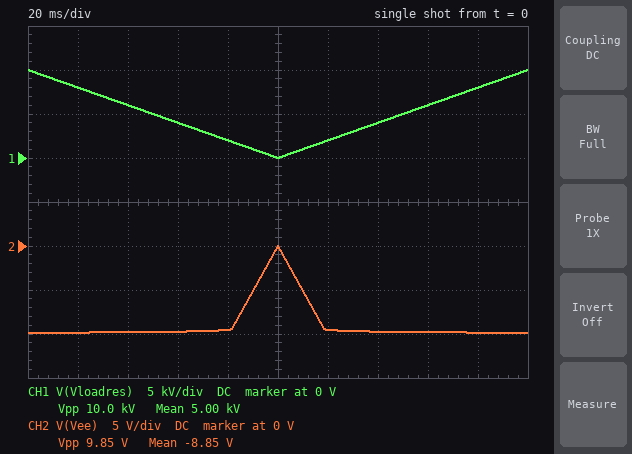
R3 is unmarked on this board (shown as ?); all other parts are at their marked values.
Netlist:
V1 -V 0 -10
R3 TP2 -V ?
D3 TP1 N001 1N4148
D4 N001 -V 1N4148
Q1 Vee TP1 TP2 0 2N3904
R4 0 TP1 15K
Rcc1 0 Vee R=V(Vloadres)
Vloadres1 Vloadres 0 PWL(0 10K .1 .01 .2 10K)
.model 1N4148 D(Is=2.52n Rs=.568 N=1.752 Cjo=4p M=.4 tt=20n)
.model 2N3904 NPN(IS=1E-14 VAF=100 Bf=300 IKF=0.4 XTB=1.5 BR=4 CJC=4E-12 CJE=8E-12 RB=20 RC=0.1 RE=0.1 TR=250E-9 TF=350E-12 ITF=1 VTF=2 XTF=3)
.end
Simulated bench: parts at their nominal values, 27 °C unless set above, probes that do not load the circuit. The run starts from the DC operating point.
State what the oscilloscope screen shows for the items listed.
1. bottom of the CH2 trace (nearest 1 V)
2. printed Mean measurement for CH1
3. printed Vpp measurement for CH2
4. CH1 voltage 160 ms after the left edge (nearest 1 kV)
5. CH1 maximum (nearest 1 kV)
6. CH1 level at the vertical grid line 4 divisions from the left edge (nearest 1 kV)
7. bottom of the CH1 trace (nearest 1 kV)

-10 V
5.00 kV
9.85 V
6 kV
10 kV
2 kV
0 V
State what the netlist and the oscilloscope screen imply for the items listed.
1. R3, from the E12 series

82 Ω
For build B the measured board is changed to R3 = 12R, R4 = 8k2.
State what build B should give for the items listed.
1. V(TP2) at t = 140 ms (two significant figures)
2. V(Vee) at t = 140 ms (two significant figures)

-10 V
-9.9 V
